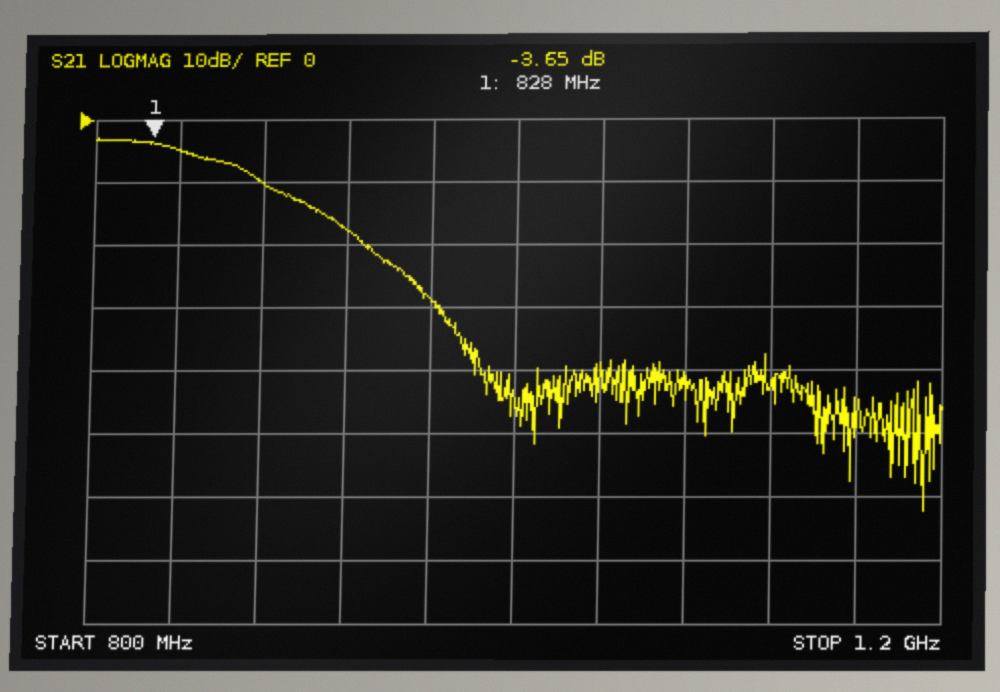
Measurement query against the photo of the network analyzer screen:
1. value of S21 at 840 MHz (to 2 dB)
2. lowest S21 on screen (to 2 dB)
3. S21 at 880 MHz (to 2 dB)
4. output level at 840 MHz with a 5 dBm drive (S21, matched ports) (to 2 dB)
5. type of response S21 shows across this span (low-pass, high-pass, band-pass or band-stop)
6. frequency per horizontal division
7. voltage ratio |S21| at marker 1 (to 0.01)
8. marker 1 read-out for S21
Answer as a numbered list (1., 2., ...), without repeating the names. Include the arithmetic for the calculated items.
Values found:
1. -4 dB
2. -62 dB
3. -10 dB
4. 5 dBm + (-4 dB) = 0 dBm
5. low-pass
6. 40 MHz
7. 10^(-3.65/20) ≈ 0.66
8. -3.65 dB
